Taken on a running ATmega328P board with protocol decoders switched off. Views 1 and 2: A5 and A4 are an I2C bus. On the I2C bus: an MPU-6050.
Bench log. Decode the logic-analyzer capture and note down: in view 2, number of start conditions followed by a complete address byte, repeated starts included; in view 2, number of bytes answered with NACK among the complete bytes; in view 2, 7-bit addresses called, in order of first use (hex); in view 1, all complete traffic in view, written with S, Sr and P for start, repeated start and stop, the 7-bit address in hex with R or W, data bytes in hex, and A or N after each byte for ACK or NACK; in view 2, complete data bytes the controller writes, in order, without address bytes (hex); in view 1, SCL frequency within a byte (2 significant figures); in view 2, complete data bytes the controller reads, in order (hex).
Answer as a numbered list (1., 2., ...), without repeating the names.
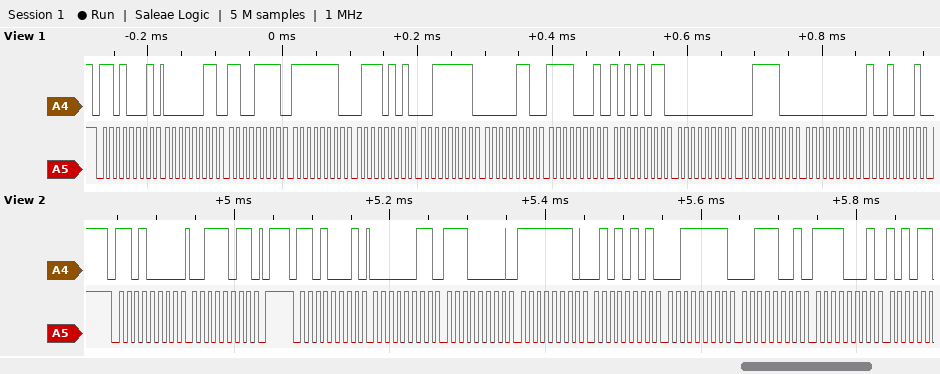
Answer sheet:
1. 2
2. 0
3. 0x68
4. S 68R A 03 A CF A FE A 75 A 3F A 06 A F1 A AB A 00 A 3C A 00 A 91 A
5. 3B
6. 100 kHz
7. 03 E0 FE 55 3F 39 F1
